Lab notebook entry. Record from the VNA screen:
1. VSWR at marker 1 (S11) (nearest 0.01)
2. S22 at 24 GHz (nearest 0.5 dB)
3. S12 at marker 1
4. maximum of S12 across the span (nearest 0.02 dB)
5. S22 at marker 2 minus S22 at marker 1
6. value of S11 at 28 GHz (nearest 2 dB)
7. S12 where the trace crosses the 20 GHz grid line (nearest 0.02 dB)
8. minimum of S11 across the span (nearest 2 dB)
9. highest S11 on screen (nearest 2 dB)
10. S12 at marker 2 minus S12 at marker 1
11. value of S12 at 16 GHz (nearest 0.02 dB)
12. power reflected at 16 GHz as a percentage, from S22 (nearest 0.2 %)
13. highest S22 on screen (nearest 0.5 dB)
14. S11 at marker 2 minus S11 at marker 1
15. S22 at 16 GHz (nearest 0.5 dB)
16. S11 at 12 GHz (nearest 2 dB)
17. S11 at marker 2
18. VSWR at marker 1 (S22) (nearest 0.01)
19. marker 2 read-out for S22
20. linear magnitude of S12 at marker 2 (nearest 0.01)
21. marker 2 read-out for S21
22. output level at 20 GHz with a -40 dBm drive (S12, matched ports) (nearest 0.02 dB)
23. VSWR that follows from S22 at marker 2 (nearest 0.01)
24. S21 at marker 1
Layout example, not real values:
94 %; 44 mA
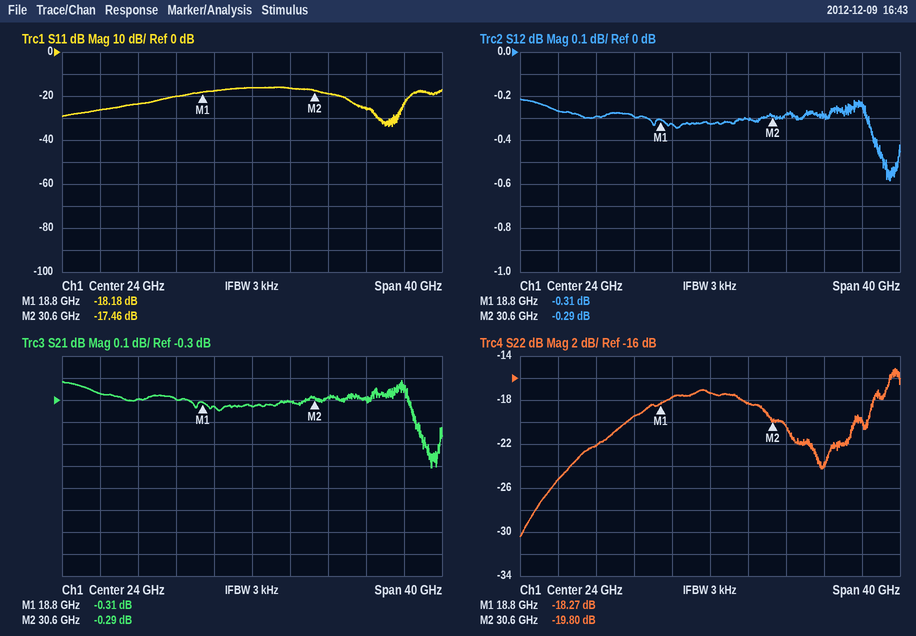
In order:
1.28; -17.5 dB; -0.31 dB; -0.22 dB; -1.53 dB; -16 dB; -0.32 dB; -34 dB; -16 dB; 0.02 dB; -0.30 dB; 1.2 %; -15.0 dB; 0.72 dB; -19.5 dB; -24 dB; -17.46 dB; 1.28; -19.80 dB; 0.97; -0.29 dB; -40.32 dBm; 1.23; -0.31 dB
